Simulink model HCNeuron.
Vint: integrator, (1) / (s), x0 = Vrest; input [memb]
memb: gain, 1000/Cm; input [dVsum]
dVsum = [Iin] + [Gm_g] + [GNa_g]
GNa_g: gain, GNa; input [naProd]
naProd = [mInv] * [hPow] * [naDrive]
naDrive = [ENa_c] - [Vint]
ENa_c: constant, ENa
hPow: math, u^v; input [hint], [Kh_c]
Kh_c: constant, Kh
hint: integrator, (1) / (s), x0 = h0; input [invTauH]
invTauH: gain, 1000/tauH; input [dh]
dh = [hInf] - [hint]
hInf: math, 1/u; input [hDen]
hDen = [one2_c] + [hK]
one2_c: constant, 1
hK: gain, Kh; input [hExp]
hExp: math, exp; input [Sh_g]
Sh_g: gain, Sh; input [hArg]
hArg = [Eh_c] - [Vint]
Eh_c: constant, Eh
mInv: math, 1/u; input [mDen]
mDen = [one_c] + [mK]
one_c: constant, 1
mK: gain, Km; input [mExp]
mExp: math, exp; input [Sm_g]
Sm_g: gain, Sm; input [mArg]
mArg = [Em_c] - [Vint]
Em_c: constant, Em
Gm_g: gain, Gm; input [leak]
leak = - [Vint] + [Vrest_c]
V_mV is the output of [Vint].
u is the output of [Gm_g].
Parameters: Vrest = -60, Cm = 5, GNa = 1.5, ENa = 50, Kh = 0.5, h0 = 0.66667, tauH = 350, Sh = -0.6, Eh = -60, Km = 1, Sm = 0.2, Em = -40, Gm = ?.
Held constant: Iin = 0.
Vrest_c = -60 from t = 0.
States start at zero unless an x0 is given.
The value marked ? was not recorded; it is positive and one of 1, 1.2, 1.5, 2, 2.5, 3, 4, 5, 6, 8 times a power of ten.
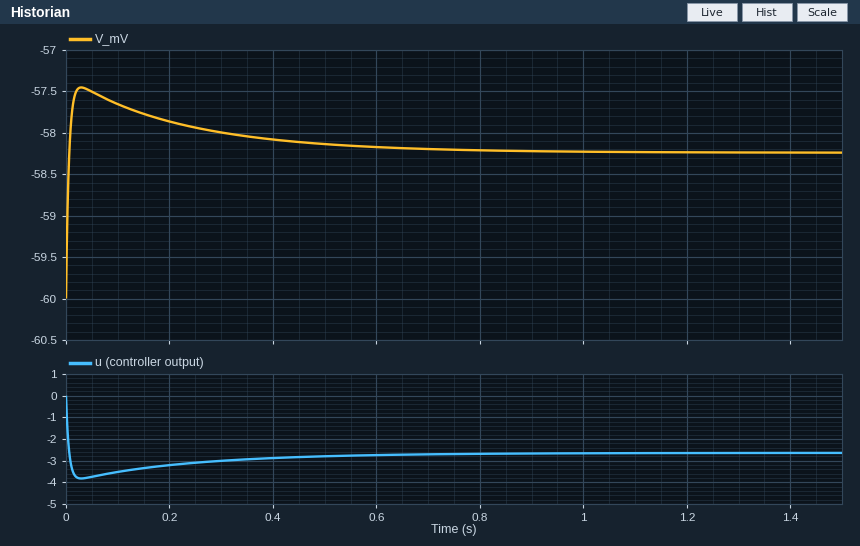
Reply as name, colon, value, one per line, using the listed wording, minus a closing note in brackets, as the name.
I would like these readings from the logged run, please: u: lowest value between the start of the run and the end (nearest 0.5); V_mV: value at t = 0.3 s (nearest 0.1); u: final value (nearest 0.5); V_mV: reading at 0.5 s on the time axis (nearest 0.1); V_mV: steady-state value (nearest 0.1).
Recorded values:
u: lowest value between the start of the run and the end: -4.0
V_mV: value at t = 0.3 s: -58.0
u: final value: -2.5
V_mV: reading at 0.5 s on the time axis: -58.1
V_mV: steady-state value: -58.2
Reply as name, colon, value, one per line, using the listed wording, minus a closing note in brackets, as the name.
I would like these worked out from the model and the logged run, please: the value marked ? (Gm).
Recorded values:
the value marked ?: 1.5
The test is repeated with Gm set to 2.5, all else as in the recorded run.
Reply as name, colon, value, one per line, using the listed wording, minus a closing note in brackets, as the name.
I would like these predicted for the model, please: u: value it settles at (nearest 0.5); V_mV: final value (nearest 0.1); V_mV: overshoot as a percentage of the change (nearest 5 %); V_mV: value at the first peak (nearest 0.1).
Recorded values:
u: value it settles at: -2.5
V_mV: final value: -59.0
V_mV: overshoot as a percentage of the change: 15 %
V_mV: value at the first peak: -58.8
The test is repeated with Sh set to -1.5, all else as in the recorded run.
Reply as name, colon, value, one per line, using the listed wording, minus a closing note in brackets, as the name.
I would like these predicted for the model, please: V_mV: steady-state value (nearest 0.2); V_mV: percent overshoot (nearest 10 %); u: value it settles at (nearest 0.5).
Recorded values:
V_mV: steady-state value: -58.8
V_mV: percent overshoot: 100 %
u: value it settles at: -2.0
